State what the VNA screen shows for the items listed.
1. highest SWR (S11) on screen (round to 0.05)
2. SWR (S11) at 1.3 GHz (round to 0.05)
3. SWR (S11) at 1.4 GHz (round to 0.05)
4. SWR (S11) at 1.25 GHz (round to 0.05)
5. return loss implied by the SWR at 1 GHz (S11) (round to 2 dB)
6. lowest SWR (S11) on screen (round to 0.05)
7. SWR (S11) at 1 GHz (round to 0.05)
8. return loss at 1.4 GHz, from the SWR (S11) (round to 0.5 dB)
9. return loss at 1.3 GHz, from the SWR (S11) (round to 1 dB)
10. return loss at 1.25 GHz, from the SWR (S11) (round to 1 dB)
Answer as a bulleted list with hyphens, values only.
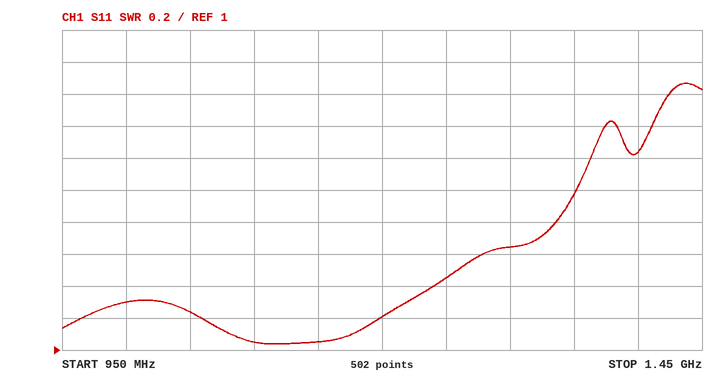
- 2.65
- 1.65
- 2.25
- 1.45
- 18 dB
- 1.05
- 1.30
- 8.5 dB
- 12 dB
- 15 dB
